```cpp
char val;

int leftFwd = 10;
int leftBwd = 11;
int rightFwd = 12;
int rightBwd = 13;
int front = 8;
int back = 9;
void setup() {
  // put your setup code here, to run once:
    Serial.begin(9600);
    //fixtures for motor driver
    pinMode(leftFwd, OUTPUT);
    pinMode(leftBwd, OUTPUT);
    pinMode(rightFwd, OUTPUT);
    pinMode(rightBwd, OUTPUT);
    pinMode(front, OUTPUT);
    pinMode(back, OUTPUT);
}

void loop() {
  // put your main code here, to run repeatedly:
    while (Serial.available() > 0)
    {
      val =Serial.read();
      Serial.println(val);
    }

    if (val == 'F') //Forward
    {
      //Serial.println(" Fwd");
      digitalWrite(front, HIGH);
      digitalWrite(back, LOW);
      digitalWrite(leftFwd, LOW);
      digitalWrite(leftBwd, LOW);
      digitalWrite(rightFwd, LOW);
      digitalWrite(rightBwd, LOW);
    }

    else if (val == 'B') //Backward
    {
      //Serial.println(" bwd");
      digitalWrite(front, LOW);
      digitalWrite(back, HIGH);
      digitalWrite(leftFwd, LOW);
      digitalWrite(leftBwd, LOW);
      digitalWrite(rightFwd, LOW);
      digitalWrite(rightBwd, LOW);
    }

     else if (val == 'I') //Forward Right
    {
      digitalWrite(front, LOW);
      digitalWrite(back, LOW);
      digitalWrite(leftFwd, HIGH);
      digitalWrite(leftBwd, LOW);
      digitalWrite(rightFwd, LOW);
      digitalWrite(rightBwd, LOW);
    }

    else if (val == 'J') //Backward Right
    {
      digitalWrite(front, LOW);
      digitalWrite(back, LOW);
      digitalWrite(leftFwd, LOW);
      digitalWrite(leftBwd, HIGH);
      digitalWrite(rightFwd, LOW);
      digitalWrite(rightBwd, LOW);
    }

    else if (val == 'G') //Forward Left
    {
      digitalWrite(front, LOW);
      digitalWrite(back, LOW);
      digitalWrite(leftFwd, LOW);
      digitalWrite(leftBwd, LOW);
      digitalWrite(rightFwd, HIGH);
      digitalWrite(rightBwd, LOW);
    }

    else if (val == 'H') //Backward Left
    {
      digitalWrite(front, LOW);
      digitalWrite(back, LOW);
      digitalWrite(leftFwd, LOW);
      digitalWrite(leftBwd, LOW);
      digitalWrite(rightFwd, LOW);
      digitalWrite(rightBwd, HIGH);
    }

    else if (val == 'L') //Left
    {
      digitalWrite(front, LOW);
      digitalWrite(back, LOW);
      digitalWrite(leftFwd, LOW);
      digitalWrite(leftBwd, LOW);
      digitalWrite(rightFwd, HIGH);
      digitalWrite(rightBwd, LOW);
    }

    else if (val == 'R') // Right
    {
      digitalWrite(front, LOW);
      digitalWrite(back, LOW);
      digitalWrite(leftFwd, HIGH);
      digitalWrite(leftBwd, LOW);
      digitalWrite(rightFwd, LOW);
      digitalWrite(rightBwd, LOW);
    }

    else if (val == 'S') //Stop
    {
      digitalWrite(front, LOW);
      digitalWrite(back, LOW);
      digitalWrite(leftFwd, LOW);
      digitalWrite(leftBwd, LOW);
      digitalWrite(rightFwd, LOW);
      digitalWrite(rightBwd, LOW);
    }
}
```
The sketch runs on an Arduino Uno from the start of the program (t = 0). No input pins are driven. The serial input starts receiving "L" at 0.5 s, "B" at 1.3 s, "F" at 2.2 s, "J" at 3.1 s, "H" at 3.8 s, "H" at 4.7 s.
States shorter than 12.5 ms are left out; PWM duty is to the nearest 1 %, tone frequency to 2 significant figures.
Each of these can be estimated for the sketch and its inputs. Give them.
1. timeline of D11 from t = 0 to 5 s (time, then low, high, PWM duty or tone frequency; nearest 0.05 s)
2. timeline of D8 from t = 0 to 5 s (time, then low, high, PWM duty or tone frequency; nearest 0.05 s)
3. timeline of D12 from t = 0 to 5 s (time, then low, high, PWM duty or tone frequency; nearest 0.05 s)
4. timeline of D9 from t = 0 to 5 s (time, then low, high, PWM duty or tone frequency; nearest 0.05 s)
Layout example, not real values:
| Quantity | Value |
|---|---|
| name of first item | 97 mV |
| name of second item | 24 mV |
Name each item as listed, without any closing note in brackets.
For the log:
| Quantity | Value |
|---|---|
| timeline of D11 from t = 0 to 5 s | 0 s low; 3.1 s high; 3.8 s low |
| timeline of D8 from t = 0 to 5 s | 0 s low; 2.2 s high; 3.1 s low |
| timeline of D12 from t = 0 to 5 s | 0 s low; 0.5 s high; 1.3 s low |
| timeline of D9 from t = 0 to 5 s | 0 s low; 1.3 s high; 2.2 s low |
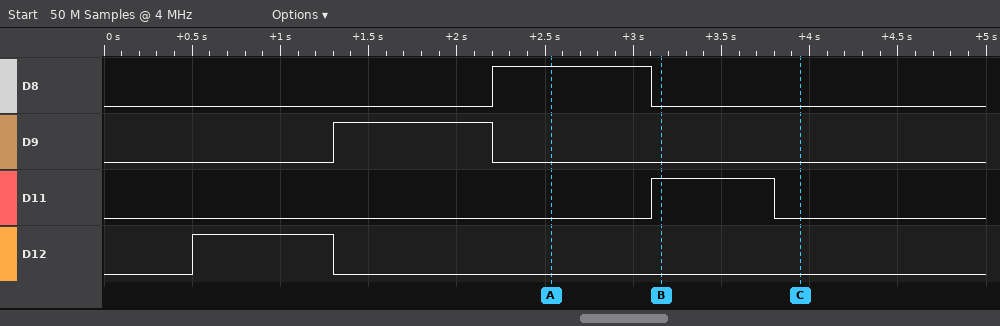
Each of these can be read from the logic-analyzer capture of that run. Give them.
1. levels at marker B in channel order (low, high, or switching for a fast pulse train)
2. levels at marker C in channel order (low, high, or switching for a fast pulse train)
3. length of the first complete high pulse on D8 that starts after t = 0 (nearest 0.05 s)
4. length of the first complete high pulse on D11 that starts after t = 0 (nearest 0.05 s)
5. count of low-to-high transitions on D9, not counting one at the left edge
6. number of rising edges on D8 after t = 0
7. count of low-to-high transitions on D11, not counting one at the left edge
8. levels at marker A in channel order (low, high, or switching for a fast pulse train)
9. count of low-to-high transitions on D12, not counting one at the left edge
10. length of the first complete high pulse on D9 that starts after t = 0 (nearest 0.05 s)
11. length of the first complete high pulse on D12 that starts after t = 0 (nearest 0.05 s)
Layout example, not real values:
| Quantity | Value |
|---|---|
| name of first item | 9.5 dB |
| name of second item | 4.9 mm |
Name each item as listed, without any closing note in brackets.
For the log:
| Quantity | Value |
|---|---|
| levels at marker B in channel order | D8 low, D9 low, D11 high, D12 low |
| levels at marker C in channel order | D8 low, D9 low, D11 low, D12 low |
| length of the first complete high pulse on D8 that starts after t = 0 | 0.90 s |
| length of the first complete high pulse on D11 that starts after t = 0 | 0.70 s |
| count of low-to-high transitions on D9, not counting one at the left edge | 1 |
| number of rising edges on D8 after t = 0 | 1 |
| count of low-to-high transitions on D11, not counting one at the left edge | 1 |
| levels at marker A in channel order | D8 high, D9 low, D11 low, D12 low |
| count of low-to-high transitions on D12, not counting one at the left edge | 1 |
| length of the first complete high pulse on D9 that starts after t = 0 | 0.90 s |
| length of the first complete high pulse on D12 that starts after t = 0 | 0.80 s |
